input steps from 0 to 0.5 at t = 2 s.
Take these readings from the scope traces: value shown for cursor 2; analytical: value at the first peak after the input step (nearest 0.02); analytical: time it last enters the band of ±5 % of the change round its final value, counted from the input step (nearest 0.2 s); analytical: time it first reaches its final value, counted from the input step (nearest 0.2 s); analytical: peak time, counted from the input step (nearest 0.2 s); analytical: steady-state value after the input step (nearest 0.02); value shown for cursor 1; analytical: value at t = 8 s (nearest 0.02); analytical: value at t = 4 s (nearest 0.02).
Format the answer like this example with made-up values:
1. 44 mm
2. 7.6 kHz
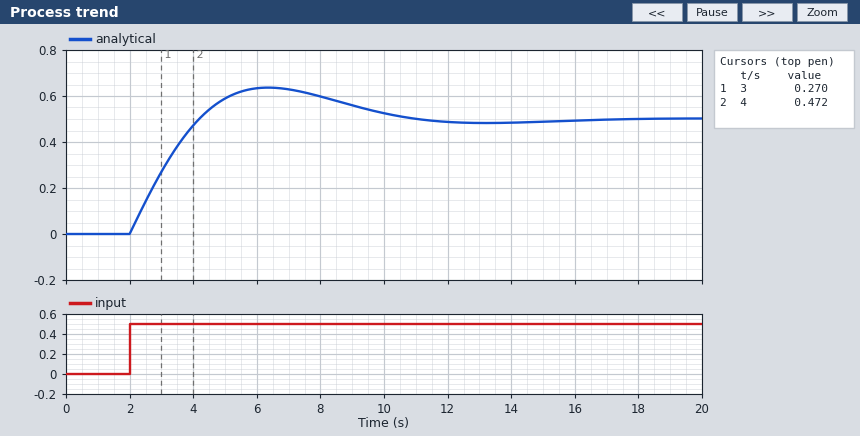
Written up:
1. 0.472
2. 0.64
3. 8.0 s
4. 2.2 s
5. 4.4 s
6. 0.50
7. 0.270
8. 0.60
9. 0.48
